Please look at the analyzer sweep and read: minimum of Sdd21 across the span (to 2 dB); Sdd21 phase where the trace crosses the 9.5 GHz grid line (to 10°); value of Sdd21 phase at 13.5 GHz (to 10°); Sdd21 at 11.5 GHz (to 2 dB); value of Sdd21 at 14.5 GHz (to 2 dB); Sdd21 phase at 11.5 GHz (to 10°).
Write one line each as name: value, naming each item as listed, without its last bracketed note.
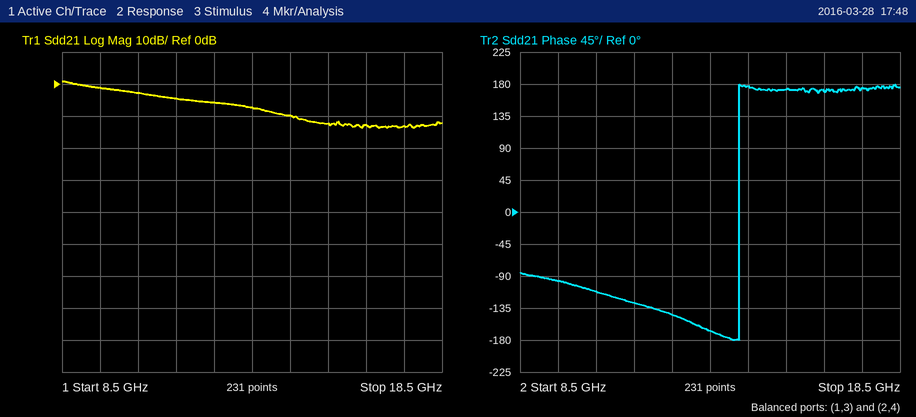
minimum of Sdd21 across the span: -14 dB
Sdd21 phase where the trace crosses the 9.5 GHz grid line: -100°
value of Sdd21 phase at 13.5 GHz: -170°
Sdd21 at 11.5 GHz: -4 dB
value of Sdd21 at 14.5 GHz: -10 dB
Sdd21 phase at 11.5 GHz: -130°
